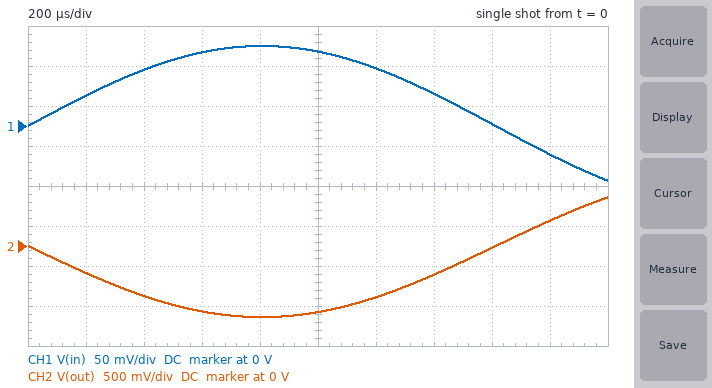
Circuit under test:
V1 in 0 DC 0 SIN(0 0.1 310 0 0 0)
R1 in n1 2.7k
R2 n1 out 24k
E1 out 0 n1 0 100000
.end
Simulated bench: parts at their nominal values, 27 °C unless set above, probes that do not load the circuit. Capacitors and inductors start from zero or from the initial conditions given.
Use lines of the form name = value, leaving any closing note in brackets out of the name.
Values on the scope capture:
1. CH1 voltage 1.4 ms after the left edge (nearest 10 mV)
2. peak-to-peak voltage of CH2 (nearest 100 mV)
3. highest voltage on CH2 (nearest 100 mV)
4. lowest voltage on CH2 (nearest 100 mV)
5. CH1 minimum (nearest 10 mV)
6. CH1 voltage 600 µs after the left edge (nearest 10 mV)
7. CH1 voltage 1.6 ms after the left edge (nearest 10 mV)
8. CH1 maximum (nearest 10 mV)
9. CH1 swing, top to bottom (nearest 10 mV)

CH1 voltage 1.4 ms after the left edge = 40 mV
peak-to-peak voltage of CH2 = 1.5 V
highest voltage on CH2 = 600 mV
lowest voltage on CH2 = -900 mV
CH1 minimum = -70 mV
CH1 voltage 600 µs after the left edge = 90 mV
CH1 voltage 1.6 ms after the left edge = 0 V
CH1 maximum = 100 mV
CH1 swing, top to bottom = 170 mV
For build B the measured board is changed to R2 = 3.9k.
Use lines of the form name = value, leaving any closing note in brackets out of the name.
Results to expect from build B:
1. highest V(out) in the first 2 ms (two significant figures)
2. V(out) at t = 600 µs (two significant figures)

highest V(out) in the first 2 ms = 99 mV
V(out) at t = 600 µs = -130 mV
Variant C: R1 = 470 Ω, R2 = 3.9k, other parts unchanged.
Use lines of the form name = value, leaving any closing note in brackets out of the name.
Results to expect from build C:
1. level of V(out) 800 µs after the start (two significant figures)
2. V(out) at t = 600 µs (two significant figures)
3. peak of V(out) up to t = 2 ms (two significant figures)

level of V(out) 800 µs after the start = -830 mV
V(out) at t = 600 µs = -760 mV
peak of V(out) up to t = 2 ms = 570 mV
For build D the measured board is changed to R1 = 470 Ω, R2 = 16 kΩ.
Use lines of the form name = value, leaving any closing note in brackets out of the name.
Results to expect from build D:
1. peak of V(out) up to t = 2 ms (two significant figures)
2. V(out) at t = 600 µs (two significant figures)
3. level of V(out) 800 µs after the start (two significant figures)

peak of V(out) up to t = 2 ms = 2.3 V
V(out) at t = 600 µs = -3.1 V
level of V(out) 800 µs after the start = -3.4 V
